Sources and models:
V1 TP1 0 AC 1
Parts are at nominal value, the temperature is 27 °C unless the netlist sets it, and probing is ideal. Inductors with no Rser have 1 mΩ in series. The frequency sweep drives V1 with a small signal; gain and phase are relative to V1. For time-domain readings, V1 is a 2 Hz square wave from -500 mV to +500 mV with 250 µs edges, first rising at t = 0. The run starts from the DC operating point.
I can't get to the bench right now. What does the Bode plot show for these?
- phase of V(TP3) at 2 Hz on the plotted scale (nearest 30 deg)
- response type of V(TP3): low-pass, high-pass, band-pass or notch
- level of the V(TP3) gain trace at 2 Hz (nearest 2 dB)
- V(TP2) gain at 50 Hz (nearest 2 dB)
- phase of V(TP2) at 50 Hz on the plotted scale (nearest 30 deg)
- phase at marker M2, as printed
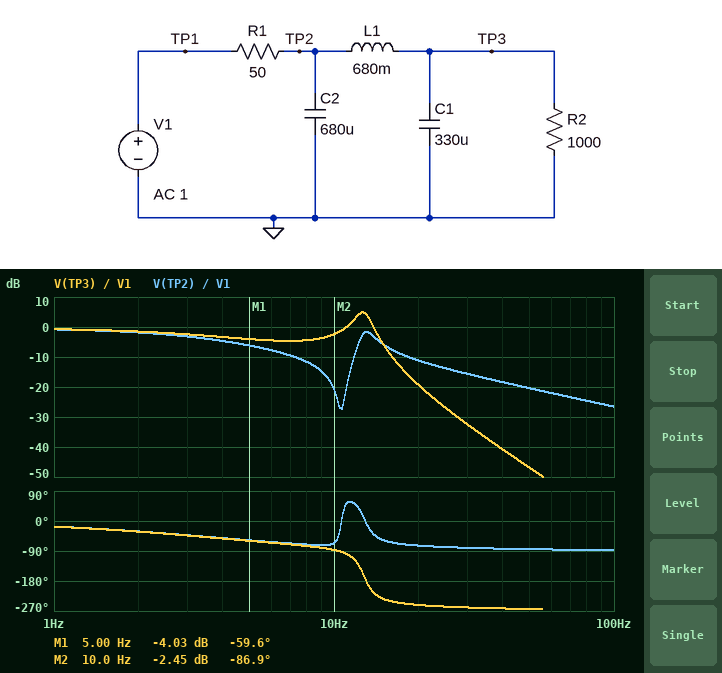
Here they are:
-30 deg
low-pass
-2 dB
-20 dB
-90 deg
-86.9 deg
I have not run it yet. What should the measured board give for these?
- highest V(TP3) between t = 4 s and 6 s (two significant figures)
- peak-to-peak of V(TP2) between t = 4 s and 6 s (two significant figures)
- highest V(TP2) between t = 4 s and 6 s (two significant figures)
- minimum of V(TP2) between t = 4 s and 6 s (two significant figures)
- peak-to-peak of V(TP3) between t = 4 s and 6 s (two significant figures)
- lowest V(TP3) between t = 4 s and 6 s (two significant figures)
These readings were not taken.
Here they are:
530 mV
990 mV
500 mV
-500 mV
1.1 V
-530 mV
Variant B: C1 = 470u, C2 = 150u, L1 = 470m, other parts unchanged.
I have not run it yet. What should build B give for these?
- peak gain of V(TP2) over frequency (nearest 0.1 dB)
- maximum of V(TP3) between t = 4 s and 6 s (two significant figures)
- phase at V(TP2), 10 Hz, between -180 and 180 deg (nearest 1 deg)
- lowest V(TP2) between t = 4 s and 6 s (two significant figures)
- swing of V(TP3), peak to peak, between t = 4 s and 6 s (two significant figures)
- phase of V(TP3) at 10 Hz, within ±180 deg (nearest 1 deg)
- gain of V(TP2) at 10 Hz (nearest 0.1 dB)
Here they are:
0 dB
480 mV
-71 deg
-480 mV
950 mV
-84 deg
-21.6 dB
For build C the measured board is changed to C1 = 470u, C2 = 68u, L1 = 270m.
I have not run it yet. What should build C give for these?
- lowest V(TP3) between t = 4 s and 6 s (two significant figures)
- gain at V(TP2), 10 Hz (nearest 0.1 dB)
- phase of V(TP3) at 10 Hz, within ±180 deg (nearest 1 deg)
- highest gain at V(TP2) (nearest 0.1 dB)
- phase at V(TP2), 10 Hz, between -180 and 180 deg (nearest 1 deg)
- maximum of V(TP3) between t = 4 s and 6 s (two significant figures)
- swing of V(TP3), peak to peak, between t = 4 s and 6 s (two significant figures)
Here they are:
-480 mV
-10.6 dB
-71 deg
0 dB
-69 deg
480 mV
950 mV
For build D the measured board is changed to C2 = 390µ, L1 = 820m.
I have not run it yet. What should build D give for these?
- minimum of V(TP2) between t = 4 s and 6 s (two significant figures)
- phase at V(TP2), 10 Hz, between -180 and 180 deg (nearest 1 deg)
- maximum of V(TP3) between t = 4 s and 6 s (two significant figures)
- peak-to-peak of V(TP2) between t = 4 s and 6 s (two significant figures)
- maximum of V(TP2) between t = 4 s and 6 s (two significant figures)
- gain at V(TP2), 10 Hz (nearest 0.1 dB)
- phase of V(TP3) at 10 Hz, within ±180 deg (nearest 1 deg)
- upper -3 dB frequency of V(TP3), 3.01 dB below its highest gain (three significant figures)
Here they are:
-510 mV
48 deg
540 mV
1.0 V
510 mV
-21.4 dB
-95 deg
13.7 Hz
